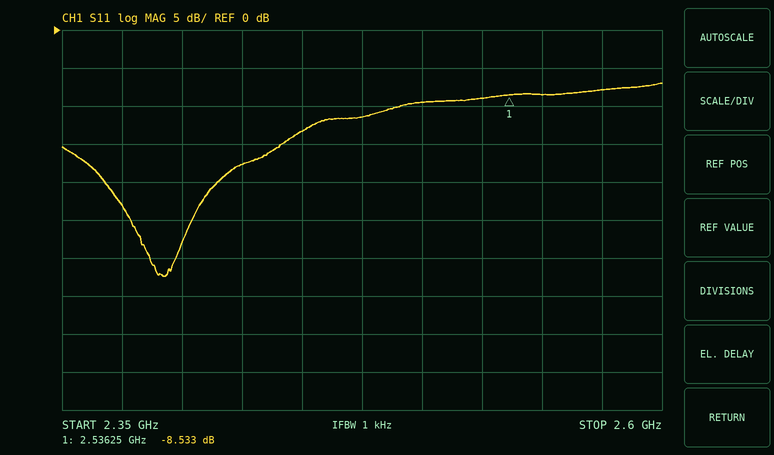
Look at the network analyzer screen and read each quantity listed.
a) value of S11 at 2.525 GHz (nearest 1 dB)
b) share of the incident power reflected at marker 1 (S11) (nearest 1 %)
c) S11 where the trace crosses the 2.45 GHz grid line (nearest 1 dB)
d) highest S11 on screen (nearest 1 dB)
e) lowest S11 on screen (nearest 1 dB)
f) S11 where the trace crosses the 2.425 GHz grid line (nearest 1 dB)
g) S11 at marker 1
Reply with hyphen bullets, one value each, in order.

- -9 dB
- 14 %
- -13 dB
- -7 dB
- -32 dB
- -18 dB
- -8.533 dB
